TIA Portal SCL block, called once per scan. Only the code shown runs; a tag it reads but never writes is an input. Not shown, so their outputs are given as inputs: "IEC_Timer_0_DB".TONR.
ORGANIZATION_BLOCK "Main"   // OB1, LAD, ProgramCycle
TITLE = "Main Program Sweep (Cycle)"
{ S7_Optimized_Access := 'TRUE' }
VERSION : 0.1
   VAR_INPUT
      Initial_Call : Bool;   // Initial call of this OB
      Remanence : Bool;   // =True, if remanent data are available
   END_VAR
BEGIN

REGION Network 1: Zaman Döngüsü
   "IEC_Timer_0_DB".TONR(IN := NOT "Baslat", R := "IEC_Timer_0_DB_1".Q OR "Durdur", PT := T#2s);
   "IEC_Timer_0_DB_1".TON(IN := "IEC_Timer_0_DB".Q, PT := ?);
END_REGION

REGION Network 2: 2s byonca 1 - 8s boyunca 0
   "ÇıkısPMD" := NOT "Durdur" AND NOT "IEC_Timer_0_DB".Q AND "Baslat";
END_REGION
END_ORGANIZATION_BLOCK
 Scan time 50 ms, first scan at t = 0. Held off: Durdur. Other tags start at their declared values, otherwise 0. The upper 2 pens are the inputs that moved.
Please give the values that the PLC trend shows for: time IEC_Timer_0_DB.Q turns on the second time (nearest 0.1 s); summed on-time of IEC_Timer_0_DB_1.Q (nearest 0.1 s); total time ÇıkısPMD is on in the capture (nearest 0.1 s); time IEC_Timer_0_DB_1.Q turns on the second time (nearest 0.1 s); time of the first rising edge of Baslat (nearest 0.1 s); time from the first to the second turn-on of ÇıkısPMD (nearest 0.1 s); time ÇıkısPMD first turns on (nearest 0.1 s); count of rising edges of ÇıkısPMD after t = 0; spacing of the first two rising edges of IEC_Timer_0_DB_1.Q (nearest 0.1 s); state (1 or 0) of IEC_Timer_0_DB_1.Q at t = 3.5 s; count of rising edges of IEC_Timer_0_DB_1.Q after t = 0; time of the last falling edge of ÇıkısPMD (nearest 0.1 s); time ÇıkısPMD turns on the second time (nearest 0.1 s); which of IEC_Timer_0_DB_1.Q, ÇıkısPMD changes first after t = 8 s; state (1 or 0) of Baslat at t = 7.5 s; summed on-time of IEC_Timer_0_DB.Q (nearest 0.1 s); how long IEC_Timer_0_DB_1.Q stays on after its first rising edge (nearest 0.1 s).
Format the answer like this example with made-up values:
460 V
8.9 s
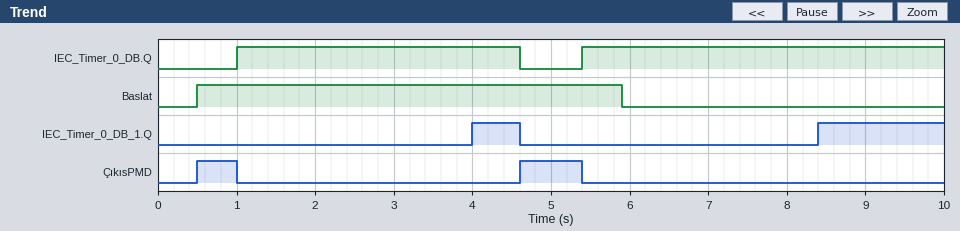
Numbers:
5.4 s
2.2 s
1.3 s
8.4 s
0.5 s
4.1 s
0.5 s
2
4.4 s
0
2
5.4 s
4.6 s
IEC_Timer_0_DB_1.Q
0
8.2 s
0.6 s
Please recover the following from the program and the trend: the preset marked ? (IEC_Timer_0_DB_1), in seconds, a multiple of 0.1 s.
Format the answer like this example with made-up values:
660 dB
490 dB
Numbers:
3.0 s
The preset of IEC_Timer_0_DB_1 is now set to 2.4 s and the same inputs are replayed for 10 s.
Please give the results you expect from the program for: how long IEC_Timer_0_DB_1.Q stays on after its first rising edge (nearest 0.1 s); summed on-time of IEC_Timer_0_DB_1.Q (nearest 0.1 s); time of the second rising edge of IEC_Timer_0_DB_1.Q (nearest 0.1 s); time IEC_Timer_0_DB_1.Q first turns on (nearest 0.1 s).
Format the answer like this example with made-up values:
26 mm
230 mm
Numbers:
1.2 s
3.4 s
7.8 s
3.4 s
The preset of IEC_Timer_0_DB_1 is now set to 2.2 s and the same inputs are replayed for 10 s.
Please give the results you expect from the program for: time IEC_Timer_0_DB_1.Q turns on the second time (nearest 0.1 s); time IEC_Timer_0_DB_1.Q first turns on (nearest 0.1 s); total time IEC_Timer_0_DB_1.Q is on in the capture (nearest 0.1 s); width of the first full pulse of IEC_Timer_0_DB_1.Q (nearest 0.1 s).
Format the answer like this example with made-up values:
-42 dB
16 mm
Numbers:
7.6 s
3.2 s
3.8 s
1.4 s
